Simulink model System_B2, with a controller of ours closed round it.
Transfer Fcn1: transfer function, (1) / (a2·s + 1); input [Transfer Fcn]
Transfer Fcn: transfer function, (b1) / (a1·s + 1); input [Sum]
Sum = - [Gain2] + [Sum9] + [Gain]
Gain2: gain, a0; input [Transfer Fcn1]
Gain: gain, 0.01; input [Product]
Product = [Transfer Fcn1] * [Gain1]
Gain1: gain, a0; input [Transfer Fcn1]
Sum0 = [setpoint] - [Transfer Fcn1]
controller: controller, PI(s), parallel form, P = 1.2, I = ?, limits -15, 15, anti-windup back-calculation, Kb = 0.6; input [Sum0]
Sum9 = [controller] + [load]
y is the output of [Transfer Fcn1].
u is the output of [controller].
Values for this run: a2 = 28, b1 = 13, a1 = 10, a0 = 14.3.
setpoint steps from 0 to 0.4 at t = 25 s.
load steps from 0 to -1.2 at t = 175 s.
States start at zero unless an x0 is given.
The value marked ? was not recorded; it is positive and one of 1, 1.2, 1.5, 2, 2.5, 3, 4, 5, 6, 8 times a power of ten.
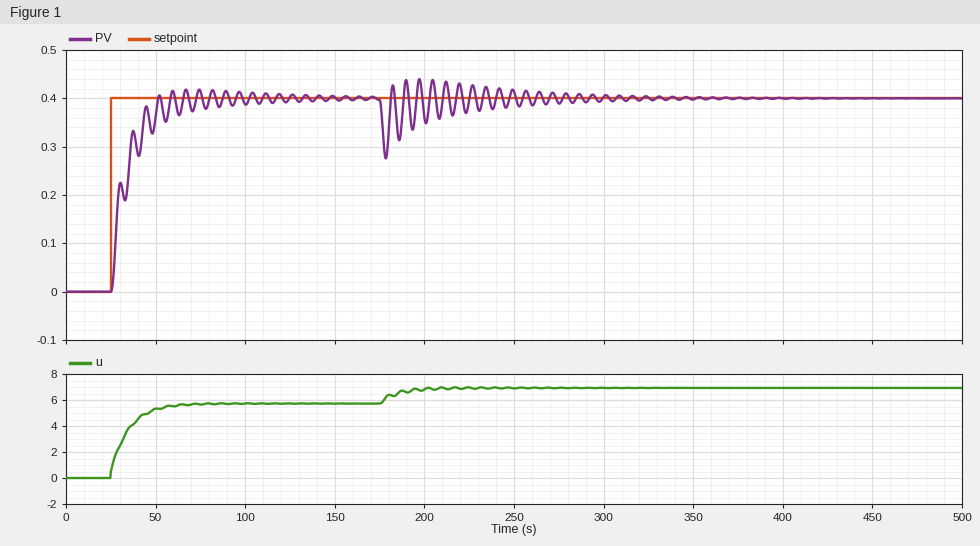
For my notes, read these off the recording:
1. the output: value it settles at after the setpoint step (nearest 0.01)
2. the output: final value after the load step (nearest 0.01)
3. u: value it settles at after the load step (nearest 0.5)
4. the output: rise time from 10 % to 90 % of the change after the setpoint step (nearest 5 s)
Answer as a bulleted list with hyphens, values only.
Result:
- 0.40
- 0.40
- 7.0
- 15 s
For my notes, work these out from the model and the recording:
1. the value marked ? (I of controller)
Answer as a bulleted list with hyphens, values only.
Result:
- 1.5
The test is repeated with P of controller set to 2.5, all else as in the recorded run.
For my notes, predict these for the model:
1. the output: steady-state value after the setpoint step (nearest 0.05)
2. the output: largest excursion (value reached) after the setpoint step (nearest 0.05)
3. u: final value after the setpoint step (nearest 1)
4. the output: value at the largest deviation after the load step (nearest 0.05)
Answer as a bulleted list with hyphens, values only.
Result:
- 0.40
- 0.40
- 6
- 0.30
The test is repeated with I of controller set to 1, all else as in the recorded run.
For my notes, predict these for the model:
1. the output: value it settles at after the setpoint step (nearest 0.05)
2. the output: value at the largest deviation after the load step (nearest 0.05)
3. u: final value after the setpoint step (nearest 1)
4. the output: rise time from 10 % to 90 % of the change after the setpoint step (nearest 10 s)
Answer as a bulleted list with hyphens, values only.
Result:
- 0.40
- 0.25
- 6
- 30 s
